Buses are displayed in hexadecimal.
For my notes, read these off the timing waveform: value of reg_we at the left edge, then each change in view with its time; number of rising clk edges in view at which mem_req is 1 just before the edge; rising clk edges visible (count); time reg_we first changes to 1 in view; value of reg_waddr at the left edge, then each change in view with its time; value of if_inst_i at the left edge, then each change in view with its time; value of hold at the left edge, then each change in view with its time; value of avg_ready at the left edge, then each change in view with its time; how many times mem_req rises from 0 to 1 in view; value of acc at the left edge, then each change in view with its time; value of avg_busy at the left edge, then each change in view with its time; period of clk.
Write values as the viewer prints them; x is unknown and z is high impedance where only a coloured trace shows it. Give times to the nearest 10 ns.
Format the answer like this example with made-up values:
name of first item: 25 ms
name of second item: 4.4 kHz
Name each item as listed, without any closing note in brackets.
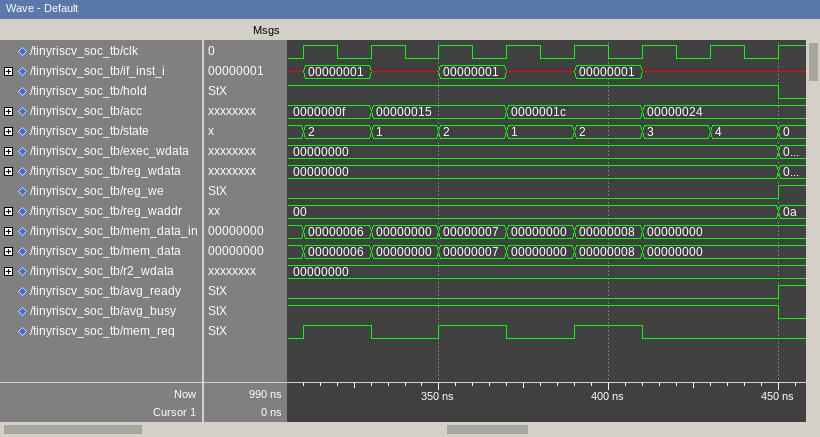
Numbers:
value of reg_we at the left edge, then each change in view with its time: 0, 1 at 450 ns
number of rising clk edges in view at which mem_req is 1 just before the edge: 3
rising clk edges visible: 8
time reg_we first changes to 1 in view: 450 ns
value of reg_waddr at the left edge, then each change in view with its time: 00, 0a at 450 ns
value of if_inst_i at the left edge, then each change in view with its time: x, 00000001 at 310 ns, x at 330 ns, 00000001 at 350 ns, x at 370 ns, 00000001 at 390 ns, x at 410 ns
value of hold at the left edge, then each change in view with its time: 1, 0 at 450 ns
value of avg_ready at the left edge, then each change in view with its time: 0, 1 at 450 ns
how many times mem_req rises from 0 to 1 in view: 3
value of acc at the left edge, then each change in view with its time: 0000000f, 00000015 at 330 ns, 0000001c at 370 ns, 00000024 at 410 ns
value of avg_busy at the left edge, then each change in view with its time: 1, 0 at 450 ns
period of clk: 20 ns
